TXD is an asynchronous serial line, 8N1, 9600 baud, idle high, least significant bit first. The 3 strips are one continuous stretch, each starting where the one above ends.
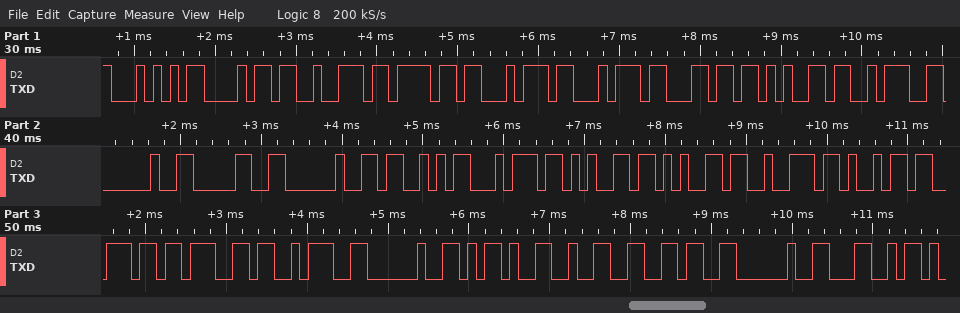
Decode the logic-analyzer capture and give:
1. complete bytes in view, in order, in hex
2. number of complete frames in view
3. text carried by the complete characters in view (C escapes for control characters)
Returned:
54 68 72 6F 74 74 6C 65 3A 20 30 20 53 74 65 65 72 69 6E 67 3A 20 2D 32 36 20 4C
27
"Throttle: 0 Steering: -26 L"
